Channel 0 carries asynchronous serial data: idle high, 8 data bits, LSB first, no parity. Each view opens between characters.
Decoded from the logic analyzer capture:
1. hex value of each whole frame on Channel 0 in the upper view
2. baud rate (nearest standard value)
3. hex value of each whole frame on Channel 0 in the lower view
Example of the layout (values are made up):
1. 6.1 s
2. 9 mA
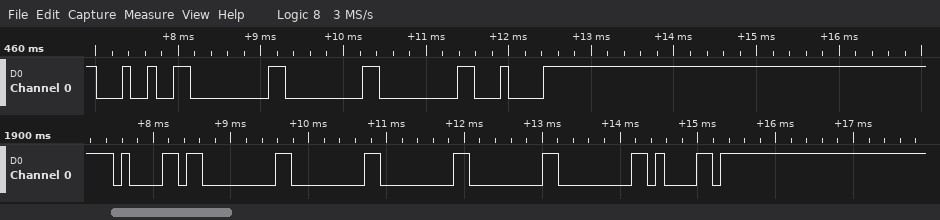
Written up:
1. 24, 00, 00, 00, 84
2. 9600 baud
3. 61, 00, 00, 00, 00, 00, 61
